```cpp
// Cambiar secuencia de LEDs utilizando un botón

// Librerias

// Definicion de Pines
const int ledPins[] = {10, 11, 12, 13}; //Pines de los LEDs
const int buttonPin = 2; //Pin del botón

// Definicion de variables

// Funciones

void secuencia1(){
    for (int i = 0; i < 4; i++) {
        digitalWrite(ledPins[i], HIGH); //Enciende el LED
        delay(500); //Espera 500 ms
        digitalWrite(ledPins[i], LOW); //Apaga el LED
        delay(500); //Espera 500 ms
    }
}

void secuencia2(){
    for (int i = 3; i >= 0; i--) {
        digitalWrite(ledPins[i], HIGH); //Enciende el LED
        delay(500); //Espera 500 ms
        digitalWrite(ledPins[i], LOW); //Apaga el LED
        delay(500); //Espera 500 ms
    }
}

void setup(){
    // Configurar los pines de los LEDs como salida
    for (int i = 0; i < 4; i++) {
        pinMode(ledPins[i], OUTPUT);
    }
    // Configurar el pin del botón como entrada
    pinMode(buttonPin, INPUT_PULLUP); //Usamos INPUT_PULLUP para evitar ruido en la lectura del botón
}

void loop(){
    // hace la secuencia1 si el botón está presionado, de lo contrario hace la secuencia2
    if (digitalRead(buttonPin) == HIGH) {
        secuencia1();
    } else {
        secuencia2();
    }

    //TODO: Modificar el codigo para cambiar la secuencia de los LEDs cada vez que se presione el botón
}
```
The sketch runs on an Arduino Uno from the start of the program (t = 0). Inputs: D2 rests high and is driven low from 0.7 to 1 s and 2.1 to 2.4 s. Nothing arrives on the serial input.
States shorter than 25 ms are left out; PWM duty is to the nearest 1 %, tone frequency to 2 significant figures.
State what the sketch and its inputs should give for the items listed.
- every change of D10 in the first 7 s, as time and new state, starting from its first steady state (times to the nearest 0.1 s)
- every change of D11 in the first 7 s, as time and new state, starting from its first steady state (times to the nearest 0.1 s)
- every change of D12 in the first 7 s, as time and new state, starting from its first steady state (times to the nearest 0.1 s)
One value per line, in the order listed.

0 s high; 0.5 s low; 4 s high; 4.5 s low
0 s low; 1 s high; 1.5 s low; 5 s high; 5.5 s low
0 s low; 2 s high; 2.5 s low; 6 s high; 6.5 s low
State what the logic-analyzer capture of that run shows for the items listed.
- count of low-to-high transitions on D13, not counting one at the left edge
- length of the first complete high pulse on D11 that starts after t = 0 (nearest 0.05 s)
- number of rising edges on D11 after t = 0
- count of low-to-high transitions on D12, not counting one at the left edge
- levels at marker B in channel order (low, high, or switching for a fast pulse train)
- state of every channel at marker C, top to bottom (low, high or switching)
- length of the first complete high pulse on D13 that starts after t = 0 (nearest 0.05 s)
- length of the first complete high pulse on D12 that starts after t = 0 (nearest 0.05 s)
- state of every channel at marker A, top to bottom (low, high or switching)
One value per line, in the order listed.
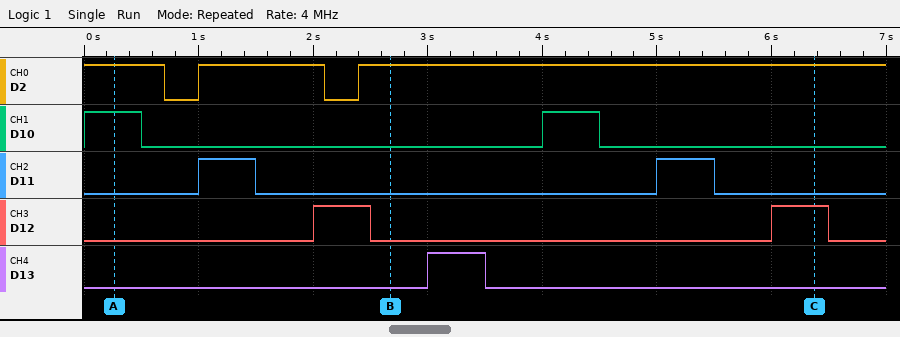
1
0.50 s
2
2
D2 high, D10 low, D11 low, D12 low, D13 low
D2 high, D10 low, D11 low, D12 high, D13 low
0.50 s
0.50 s
D2 high, D10 high, D11 low, D12 low, D13 low
